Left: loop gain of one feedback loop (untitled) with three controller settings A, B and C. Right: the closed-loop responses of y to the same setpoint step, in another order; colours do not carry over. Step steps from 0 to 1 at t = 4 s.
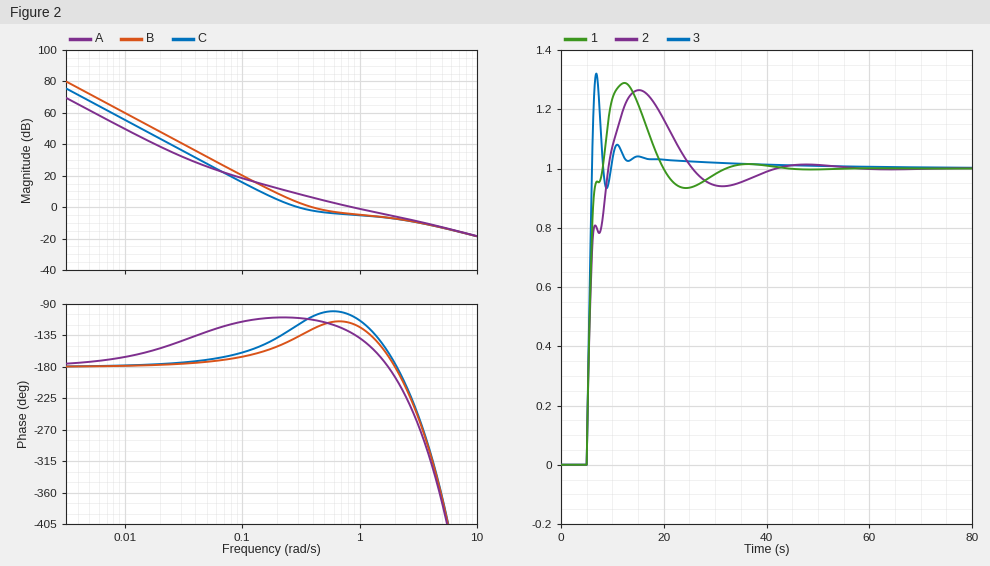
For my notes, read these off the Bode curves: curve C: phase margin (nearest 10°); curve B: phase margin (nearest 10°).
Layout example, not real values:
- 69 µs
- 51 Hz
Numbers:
- 60°
- 50°
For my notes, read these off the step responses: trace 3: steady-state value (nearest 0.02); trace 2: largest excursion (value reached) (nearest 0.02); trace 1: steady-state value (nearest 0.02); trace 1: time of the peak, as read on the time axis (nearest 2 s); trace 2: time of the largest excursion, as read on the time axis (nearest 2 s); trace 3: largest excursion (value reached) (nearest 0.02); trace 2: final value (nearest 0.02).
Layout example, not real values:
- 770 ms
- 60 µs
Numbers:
- 1.00
- 1.26
- 1.00
- 12 s
- 16 s
- 1.32
- 1.00
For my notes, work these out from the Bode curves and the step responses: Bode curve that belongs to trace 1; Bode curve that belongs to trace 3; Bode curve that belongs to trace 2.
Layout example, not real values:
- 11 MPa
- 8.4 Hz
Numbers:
- B
- A
- C
